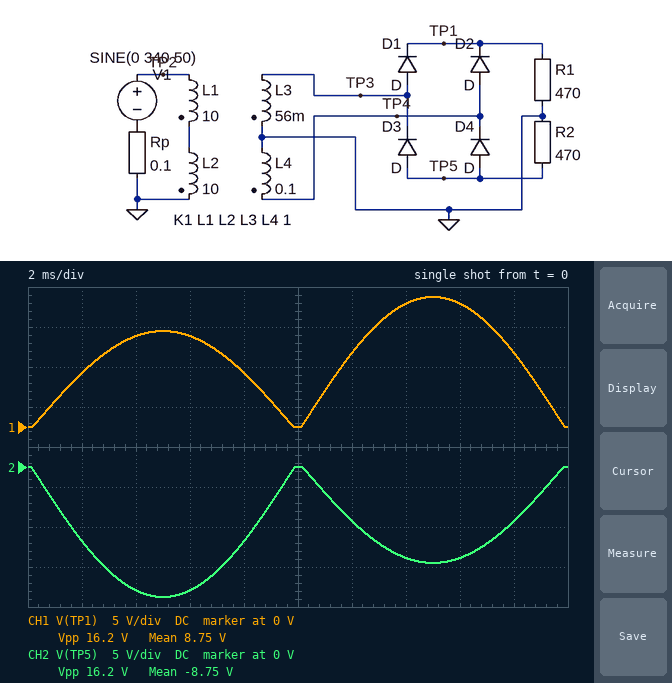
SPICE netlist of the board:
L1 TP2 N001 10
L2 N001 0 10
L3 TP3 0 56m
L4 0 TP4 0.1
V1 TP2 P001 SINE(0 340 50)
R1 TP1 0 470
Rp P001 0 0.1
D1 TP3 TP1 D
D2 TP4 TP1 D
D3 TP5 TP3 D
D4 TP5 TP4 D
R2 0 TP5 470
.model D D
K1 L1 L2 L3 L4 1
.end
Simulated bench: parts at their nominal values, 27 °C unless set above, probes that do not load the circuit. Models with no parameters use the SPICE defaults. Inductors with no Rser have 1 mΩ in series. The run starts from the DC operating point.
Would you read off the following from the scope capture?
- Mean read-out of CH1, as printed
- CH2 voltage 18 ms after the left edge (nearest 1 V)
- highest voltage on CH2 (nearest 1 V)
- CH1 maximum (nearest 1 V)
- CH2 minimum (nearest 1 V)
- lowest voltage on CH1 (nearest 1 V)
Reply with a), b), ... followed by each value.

a) 8.75 V
b) -7 V
c) 0 V
d) 16 V
e) -16 V
f) 0 V
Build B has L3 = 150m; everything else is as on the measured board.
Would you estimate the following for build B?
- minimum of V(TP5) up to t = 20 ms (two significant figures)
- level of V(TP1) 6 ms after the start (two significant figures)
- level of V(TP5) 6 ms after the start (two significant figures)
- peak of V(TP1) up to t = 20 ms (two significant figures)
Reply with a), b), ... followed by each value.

a) -20 V
b) 19 V
c) -15 V
d) 20 V
